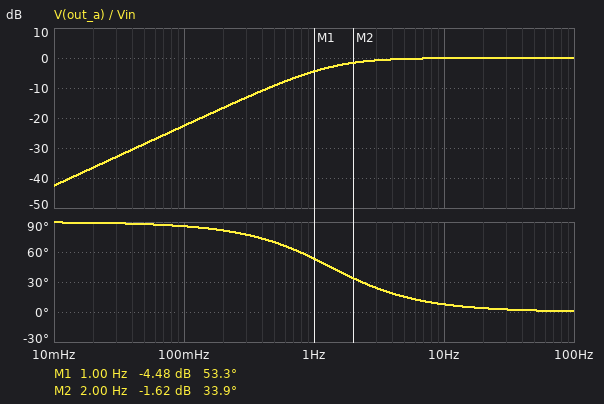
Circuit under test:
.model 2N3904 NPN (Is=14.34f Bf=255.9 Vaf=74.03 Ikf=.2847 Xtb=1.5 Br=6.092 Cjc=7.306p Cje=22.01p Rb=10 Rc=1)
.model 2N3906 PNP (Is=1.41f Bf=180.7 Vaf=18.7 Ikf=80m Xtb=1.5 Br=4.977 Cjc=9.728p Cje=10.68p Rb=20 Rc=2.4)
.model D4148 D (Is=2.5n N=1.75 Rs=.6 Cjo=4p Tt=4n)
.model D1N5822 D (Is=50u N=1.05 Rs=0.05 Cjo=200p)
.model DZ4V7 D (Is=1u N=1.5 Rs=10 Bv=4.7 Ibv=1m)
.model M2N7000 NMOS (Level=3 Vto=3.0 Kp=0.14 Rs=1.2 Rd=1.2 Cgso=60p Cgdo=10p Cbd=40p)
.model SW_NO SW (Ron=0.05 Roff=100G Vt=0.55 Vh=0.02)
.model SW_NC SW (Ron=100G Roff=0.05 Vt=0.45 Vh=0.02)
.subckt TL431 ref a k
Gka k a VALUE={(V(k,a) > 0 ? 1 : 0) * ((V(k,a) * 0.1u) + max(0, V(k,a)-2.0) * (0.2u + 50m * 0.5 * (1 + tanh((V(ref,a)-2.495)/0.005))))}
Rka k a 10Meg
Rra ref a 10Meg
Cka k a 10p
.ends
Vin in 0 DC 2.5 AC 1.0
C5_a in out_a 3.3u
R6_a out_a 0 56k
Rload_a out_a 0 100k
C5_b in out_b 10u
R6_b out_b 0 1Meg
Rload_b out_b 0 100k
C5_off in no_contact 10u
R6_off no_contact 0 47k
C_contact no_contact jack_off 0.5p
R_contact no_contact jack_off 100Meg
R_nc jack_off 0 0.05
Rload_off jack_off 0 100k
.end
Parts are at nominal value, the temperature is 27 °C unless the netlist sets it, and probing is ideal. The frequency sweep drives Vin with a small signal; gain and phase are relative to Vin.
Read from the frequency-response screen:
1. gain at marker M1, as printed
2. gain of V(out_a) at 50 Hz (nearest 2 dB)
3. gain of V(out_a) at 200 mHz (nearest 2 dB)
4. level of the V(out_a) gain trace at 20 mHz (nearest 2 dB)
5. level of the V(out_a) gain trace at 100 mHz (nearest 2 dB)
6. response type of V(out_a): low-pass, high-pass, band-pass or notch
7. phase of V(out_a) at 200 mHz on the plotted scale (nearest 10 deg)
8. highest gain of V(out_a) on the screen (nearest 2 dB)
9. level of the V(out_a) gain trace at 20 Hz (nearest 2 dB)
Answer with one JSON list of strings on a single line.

["-4.48 dB", "0 dB", "-16 dB", "-36 dB", "-22 dB", "high-pass", "80 deg", "0 dB", "0 dB"]
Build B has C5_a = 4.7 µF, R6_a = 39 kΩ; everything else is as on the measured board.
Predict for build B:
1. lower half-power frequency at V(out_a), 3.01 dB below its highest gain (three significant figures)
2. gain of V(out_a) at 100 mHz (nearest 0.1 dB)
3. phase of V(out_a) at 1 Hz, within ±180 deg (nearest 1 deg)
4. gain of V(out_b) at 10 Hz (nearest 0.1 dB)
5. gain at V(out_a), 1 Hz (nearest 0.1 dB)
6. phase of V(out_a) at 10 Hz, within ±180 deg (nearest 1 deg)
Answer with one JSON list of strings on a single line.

["1.21 Hz", "-21.7 dB", "50 deg", "0 dB", "-3.9 dB", "7 deg"]
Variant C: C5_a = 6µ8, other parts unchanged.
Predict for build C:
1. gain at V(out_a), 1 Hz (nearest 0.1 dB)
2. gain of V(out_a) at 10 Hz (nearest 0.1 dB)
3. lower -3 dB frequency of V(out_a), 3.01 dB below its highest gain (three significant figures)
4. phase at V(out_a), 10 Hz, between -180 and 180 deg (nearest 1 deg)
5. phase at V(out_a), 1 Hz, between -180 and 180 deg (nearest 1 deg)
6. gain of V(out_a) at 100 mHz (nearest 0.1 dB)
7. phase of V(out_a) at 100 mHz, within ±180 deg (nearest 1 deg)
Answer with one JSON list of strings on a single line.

["-1.5 dB", "0 dB", "652 mHz", "4 deg", "33 deg", "-16.4 dB", "81 deg"]
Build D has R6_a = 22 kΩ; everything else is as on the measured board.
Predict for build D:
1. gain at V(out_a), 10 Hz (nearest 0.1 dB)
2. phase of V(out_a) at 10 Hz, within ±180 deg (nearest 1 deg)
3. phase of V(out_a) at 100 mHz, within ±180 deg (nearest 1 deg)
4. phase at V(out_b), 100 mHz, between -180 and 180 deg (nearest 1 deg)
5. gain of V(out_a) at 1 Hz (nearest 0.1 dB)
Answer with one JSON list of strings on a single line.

["-0.3 dB", "15 deg", "88 deg", "60 deg", "-9.1 dB"]
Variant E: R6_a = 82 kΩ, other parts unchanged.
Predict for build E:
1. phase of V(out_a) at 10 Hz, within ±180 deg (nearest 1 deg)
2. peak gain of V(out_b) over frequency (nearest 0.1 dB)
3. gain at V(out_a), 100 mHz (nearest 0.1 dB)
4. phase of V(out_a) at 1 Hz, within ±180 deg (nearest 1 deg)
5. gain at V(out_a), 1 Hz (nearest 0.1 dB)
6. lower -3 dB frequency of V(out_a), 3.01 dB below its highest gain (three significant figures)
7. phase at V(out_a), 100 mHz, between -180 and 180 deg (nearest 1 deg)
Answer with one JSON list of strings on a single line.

["6 deg", "0 dB", "-20.6 dB", "47 deg", "-3.3 dB", "1.07 Hz", "85 deg"]
